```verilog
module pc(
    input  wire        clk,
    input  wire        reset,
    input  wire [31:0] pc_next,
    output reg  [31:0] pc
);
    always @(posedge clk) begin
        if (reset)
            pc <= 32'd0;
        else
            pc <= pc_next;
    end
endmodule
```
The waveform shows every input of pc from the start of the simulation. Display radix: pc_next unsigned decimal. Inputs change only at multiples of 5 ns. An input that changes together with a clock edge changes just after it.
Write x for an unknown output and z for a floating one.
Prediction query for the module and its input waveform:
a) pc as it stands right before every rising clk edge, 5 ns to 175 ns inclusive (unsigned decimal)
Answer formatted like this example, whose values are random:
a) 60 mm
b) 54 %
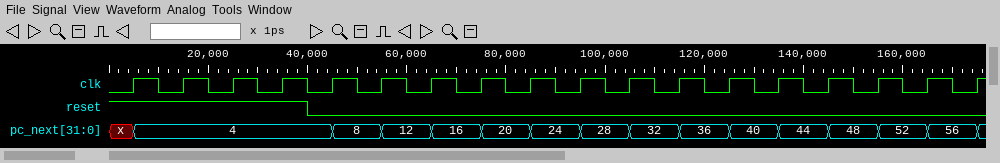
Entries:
a) x, 0, 0, 0, 0, 4, 8, 12, 16, 20, 24, 28, 32, 36, 40, 44, 48, 52
